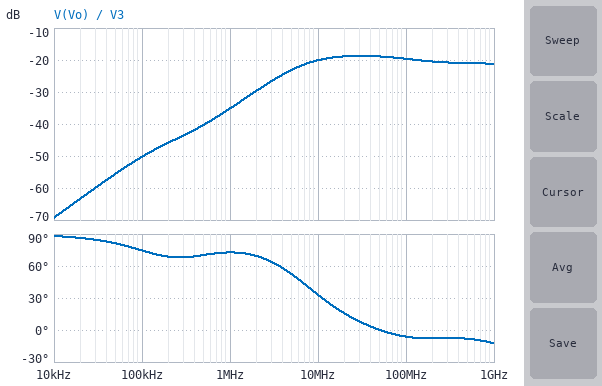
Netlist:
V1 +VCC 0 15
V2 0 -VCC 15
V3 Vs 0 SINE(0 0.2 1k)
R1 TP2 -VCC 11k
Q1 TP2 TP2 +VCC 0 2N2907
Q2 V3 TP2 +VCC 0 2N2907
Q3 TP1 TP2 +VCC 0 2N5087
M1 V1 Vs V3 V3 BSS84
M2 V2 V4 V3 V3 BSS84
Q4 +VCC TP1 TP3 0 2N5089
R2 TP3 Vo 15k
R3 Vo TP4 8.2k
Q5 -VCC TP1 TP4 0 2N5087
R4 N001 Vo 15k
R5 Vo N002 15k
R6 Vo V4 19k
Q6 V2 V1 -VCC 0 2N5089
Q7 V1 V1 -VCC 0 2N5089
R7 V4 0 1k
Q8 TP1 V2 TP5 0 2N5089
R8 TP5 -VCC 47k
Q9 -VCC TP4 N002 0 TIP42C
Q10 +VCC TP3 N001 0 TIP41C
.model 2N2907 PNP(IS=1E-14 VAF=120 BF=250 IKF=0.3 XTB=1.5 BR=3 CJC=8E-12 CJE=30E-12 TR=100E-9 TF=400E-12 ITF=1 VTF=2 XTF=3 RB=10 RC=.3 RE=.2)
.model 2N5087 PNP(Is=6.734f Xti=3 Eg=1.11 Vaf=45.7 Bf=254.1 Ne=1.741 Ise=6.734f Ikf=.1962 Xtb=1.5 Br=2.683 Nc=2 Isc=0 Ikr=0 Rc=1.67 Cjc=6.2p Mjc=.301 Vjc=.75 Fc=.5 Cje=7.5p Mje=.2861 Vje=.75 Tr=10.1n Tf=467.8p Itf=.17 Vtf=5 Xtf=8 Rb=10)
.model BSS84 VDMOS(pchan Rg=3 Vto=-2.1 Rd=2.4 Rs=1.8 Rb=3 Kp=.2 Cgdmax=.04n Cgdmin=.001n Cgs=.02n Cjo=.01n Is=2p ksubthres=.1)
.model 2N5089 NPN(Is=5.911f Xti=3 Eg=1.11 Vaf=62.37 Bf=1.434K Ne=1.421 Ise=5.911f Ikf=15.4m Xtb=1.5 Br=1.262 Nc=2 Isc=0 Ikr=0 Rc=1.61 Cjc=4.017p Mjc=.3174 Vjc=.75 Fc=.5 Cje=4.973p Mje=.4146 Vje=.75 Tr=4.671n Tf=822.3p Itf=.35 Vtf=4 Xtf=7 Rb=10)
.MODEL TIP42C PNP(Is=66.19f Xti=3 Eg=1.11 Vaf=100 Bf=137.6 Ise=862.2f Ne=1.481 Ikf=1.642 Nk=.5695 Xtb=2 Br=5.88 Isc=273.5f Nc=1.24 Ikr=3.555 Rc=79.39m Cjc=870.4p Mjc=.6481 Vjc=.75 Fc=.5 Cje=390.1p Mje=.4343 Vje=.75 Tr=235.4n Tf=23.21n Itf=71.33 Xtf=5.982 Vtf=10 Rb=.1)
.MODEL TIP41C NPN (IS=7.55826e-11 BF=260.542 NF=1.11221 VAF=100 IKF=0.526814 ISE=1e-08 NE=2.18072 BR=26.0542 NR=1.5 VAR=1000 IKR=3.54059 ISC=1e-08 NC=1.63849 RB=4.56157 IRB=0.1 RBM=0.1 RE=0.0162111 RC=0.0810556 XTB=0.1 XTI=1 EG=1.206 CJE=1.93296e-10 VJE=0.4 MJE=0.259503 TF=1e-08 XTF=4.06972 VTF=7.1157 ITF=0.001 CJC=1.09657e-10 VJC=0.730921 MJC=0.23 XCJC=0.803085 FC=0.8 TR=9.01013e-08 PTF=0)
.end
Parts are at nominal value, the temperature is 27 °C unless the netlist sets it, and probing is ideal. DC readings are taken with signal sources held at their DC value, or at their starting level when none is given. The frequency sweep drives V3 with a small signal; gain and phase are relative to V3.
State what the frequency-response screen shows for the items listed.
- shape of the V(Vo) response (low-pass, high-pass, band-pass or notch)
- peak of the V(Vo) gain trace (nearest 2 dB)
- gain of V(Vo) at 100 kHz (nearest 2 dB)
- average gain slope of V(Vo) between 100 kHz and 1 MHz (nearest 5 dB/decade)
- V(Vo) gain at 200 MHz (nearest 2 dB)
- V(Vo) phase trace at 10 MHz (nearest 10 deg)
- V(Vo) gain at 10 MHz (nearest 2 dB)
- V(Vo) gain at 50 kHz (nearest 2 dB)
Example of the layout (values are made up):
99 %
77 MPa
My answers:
high-pass
-18 dB
-50 dB
15 dB/decade
-20 dB
30 deg
-20 dB
-56 dB
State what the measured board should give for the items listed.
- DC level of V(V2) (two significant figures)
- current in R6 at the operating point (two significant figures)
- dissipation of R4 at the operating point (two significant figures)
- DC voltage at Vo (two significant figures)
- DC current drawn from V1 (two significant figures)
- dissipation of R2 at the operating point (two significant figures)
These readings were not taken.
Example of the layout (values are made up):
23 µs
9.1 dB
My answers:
-15 V
510 µA
880 µW
10 V
5.7 mA
1.1 mW
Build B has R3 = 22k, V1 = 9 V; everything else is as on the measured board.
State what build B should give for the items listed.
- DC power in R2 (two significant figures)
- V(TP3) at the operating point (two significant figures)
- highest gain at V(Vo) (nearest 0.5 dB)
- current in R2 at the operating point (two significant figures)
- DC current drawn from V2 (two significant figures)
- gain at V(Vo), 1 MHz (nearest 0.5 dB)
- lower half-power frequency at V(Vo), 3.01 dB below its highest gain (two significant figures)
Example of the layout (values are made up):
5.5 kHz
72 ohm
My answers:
390 µW
8.4 V
-17.0 dB
160 µA
4.0 mA
-33.5 dB
6.4 MHz
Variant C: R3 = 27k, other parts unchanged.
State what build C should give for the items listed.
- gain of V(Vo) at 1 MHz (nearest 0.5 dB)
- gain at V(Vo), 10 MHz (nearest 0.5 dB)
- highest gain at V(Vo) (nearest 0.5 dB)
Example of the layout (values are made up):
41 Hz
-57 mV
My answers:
-33.0 dB
-18.0 dB
-16.5 dB
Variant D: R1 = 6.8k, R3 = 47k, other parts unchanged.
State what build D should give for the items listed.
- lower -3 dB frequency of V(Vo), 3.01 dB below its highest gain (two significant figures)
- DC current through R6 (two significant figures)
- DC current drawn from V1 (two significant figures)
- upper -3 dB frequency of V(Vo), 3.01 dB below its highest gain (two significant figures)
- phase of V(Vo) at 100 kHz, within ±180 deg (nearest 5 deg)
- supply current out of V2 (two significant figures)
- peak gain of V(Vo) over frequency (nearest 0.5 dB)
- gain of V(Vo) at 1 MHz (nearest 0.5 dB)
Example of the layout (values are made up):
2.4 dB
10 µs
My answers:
6.6 MHz
510 µA
8.9 mA
1.5 GHz
80 deg
8.4 mA
-16.0 dB
-32.5 dB
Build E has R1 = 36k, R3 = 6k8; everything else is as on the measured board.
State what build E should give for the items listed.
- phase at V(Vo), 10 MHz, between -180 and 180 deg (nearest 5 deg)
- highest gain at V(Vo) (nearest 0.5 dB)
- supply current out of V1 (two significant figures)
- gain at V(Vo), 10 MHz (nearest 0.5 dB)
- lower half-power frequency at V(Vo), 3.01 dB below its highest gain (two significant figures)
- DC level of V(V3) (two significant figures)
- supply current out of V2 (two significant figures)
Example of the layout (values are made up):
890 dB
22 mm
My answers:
30 deg
-20.0 dB
2.1 mA
-21.0 dB
5.8 MHz
2.1 V
1.6 mA
